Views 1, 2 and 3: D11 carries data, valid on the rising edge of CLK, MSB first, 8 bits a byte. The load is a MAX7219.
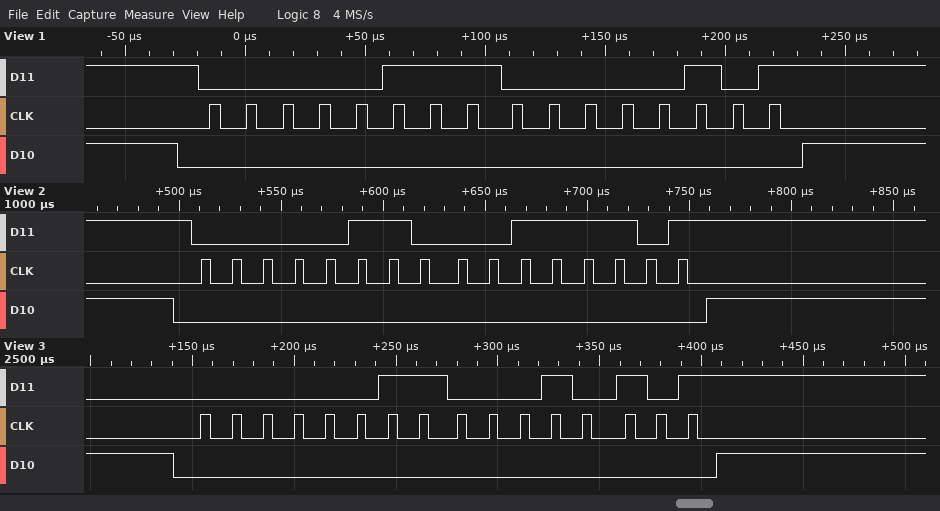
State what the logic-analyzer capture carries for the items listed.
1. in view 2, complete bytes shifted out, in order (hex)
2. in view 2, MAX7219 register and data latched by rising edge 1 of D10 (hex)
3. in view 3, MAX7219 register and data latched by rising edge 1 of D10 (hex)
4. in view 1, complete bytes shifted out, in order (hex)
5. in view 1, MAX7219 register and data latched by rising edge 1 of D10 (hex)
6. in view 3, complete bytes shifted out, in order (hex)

0x06 0x3D
register 0x6, data 0x3D
register 0x3, data 0x15
07 05
register 0x7, data 0x05
0x03 0x15
